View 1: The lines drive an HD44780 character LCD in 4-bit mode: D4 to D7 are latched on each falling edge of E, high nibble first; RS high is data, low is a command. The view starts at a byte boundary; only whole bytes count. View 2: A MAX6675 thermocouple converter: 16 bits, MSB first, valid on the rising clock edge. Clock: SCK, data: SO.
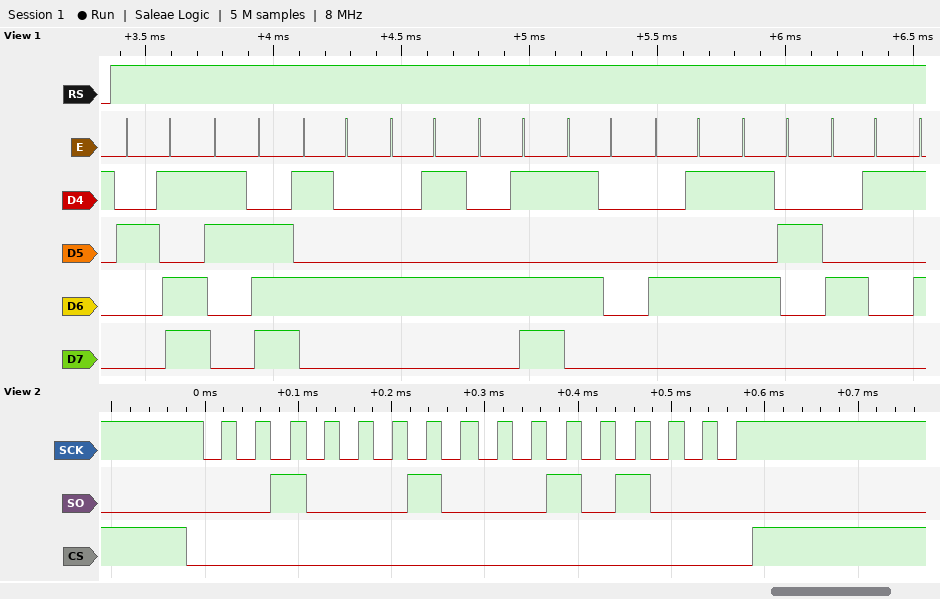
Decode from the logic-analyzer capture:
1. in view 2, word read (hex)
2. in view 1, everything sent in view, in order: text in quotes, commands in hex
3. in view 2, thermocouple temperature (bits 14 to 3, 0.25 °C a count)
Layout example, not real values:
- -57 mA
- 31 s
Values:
- 0x2228
- "->TEMPERA"
- 273.25 °C
